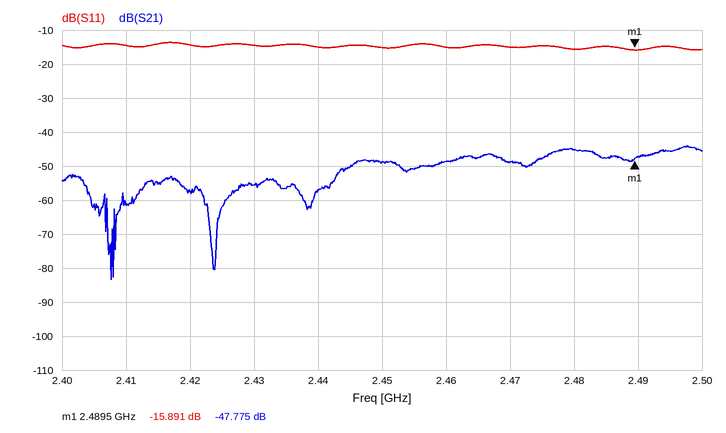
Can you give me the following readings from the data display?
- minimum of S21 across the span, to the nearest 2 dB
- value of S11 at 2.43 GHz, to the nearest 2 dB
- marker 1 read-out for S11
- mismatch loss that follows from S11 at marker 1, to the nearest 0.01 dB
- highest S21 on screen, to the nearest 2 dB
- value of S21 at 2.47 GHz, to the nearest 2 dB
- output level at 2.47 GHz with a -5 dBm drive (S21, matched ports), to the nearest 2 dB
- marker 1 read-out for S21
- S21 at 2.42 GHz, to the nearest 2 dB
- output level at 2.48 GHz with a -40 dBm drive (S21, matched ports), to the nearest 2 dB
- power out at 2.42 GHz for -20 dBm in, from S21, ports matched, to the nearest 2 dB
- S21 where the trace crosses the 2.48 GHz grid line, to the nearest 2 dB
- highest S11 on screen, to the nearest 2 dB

-84 dB
-14 dB
-15.891 dB
0.11 dB
-44 dB
-48 dB
-54 dBm
-47.775 dB
-58 dB
-86 dBm
-78 dBm
-46 dB
-14 dB
